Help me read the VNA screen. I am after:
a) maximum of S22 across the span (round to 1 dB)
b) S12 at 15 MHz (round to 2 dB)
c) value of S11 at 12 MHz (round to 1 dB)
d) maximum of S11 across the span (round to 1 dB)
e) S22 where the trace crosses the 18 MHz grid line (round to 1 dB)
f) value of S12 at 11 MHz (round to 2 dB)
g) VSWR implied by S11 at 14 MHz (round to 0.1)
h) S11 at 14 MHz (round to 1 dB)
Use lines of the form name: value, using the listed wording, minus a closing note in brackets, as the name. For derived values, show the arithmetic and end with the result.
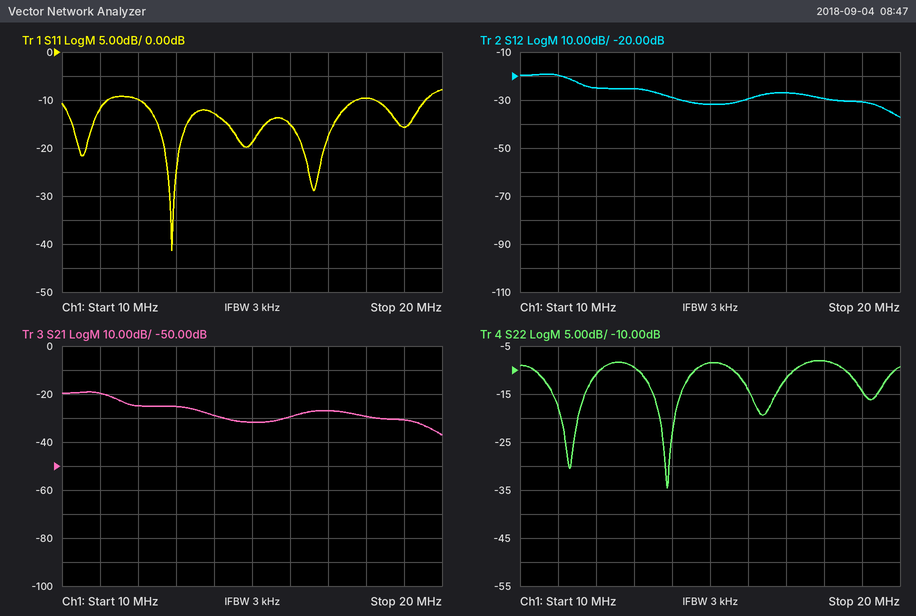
maximum of S22 across the span: -8 dB
S12 at 15 MHz: -32 dB
value of S11 at 12 MHz: -10 dB
maximum of S11 across the span: -8 dB
S22 where the trace crosses the 18 MHz grid line: -8 dB
value of S12 at 11 MHz: -20 dB
VSWR implied by S11 at 14 MHz: |Γ| = 10^(-13/20) = 0.2239; VSWR = (1 + 0.2239)/(1 − 0.2239) ≈ 1.6
S11 at 14 MHz: -13 dB
